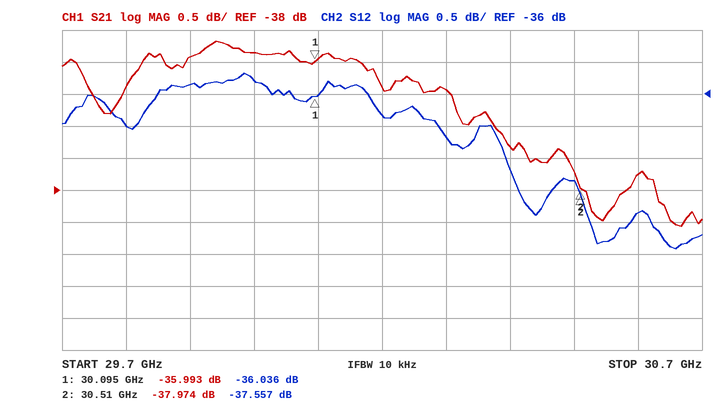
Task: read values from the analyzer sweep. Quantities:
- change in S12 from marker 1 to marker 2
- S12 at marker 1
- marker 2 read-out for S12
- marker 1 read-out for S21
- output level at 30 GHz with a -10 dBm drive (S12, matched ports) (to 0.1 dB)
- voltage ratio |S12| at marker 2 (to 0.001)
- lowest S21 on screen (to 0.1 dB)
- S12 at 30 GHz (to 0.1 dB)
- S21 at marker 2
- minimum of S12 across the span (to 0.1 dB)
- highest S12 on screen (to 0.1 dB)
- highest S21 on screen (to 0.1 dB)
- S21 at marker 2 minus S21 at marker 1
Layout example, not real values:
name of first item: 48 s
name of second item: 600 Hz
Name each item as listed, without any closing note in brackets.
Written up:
change in S12 from marker 1 to marker 2: -1.521 dB
S12 at marker 1: -36.036 dB
marker 2 read-out for S12: -37.557 dB
marker 1 read-out for S21: -35.993 dB
output level at 30 GHz with a -10 dBm drive (S12, matched ports): -45.8 dBm
voltage ratio |S12| at marker 2: 0.013
lowest S21 on screen: -38.6 dB
S12 at 30 GHz: -35.8 dB
S21 at marker 2: -37.974 dB
minimum of S12 across the span: -38.4 dB
highest S12 on screen: -35.7 dB
highest S21 on screen: -35.7 dB
S21 at marker 2 minus S21 at marker 1: -1.981 dB
